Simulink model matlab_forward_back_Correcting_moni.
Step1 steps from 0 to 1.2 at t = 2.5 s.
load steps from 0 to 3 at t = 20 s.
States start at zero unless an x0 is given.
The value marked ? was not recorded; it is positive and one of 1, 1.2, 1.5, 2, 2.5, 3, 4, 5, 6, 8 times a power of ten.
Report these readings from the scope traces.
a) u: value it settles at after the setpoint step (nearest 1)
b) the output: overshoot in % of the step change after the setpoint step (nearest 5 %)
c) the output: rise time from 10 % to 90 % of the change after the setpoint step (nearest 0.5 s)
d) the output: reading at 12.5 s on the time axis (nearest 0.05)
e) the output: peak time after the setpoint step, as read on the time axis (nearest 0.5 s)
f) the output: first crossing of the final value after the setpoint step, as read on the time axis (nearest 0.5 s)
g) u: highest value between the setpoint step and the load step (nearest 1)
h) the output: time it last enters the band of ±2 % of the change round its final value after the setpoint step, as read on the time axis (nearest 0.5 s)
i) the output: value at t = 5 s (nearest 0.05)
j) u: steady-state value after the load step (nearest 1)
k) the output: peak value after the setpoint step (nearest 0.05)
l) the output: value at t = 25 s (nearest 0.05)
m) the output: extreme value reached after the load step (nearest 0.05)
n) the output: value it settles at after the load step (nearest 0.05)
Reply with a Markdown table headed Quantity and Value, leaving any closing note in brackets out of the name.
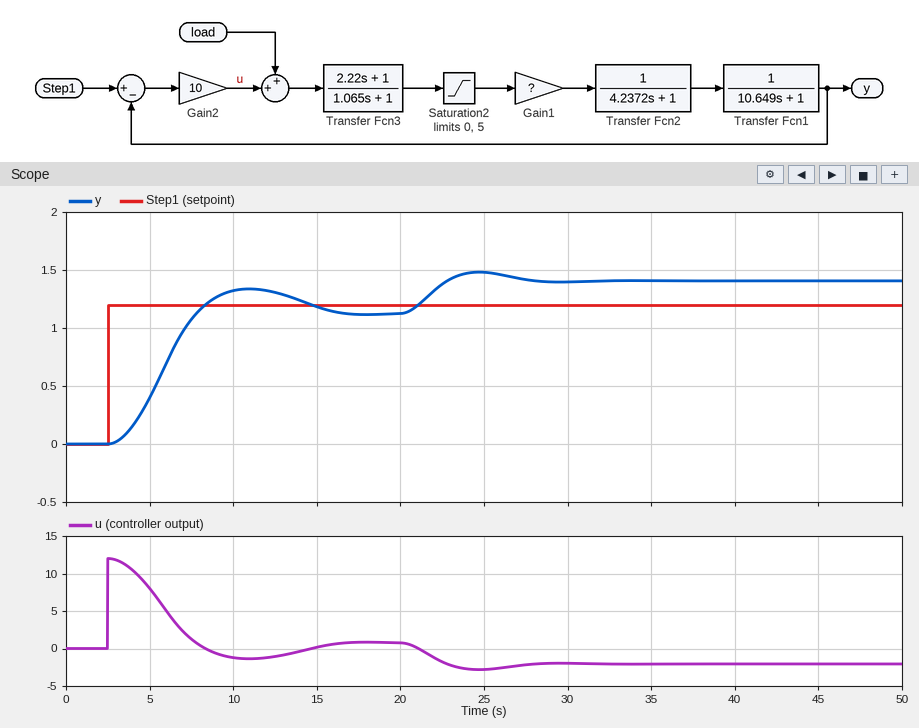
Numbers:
| Quantity | Value |
|---|---|
| u: value it settles at after the setpoint step | 1 |
| the output: overshoot in % of the step change after the setpoint step | 20 % |
| the output: rise time from 10 % to 90 % of the change after the setpoint step | 3.5 s |
| the output: reading at 12.5 s on the time axis | 1.30 |
| the output: peak time after the setpoint step, as read on the time axis | 11.0 s |
| the output: first crossing of the final value after the setpoint step, as read on the time axis | 8.0 s |
| u: highest value between the setpoint step and the load step | 12 |
| the output: time it last enters the band of ±2 % of the change round its final value after the setpoint step, as read on the time axis | 16.0 s |
| the output: value at t = 5 s | 0.40 |
| u: steady-state value after the load step | -2 |
| the output: peak value after the setpoint step | 1.35 |
| the output: value at t = 25 s | 1.50 |
| the output: extreme value reached after the load step | 1.50 |
| the output: value it settles at after the load step | 1.40 |
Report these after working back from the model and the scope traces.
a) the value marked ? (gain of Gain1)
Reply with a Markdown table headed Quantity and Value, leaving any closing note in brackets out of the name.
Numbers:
| Quantity | Value |
|---|---|
| the value marked ? | 1.5 |
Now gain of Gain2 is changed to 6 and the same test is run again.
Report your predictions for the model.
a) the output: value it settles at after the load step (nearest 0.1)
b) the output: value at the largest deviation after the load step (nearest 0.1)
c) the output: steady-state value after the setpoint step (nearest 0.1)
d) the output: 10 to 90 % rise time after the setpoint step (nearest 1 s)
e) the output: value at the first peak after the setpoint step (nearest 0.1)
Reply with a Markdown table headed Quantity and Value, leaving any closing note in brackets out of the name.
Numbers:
| Quantity | Value |
|---|---|
| the output: value it settles at after the load step | 1.5 |
| the output: value at the largest deviation after the load step | 1.6 |
| the output: steady-state value after the setpoint step | 1.1 |
| the output: 10 to 90 % rise time after the setpoint step | 4 s |
| the output: value at the first peak after the setpoint step | 1.2 |
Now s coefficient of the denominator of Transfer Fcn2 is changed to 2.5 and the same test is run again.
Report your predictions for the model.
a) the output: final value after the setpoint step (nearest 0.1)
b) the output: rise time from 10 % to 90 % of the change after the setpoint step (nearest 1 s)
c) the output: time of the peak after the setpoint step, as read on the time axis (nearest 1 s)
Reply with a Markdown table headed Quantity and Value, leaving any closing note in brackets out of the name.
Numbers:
| Quantity | Value |
|---|---|
| the output: final value after the setpoint step | 1.1 |
| the output: rise time from 10 % to 90 % of the change after the setpoint step | 3 s |
| the output: time of the peak after the setpoint step, as read on the time axis | 9 s |
